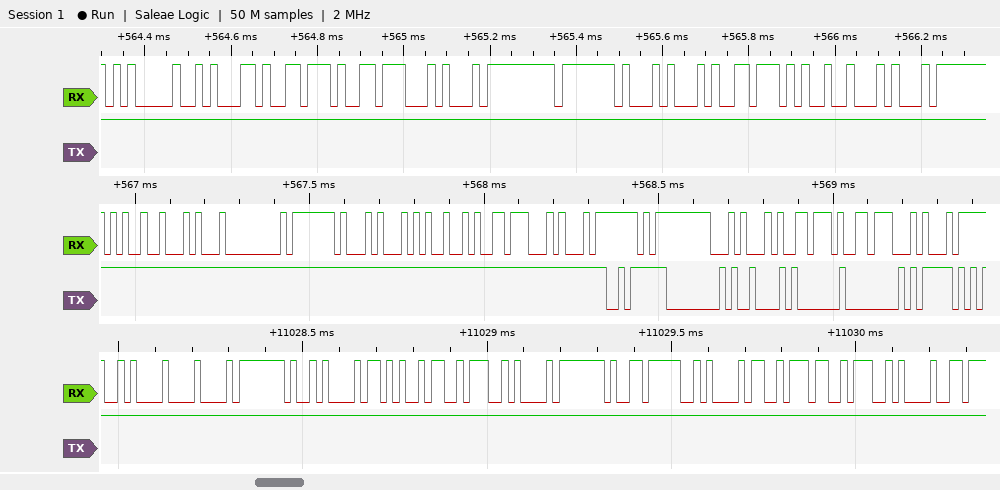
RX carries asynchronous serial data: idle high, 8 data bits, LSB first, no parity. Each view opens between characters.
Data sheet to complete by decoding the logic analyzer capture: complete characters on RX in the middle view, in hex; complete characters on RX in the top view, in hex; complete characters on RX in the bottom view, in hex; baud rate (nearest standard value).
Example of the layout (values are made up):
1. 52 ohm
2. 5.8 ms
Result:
1. 25, 14, 00, 7F, 14, 25, D9, 14, 7F, FF, 14, D9, D9, 14
2. 05, 8A, D9, D9, 14, FF, 7F, 14, D9, 25, 14
3. 0A, 08, 7F, 0A, 2B, D3, 0A, 7F, F6, 0A, D3, D3, 0A
4. 57600 baud
